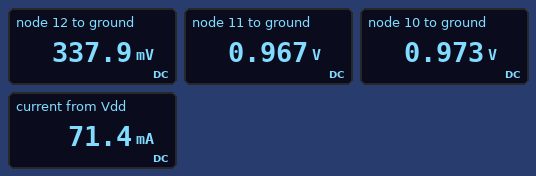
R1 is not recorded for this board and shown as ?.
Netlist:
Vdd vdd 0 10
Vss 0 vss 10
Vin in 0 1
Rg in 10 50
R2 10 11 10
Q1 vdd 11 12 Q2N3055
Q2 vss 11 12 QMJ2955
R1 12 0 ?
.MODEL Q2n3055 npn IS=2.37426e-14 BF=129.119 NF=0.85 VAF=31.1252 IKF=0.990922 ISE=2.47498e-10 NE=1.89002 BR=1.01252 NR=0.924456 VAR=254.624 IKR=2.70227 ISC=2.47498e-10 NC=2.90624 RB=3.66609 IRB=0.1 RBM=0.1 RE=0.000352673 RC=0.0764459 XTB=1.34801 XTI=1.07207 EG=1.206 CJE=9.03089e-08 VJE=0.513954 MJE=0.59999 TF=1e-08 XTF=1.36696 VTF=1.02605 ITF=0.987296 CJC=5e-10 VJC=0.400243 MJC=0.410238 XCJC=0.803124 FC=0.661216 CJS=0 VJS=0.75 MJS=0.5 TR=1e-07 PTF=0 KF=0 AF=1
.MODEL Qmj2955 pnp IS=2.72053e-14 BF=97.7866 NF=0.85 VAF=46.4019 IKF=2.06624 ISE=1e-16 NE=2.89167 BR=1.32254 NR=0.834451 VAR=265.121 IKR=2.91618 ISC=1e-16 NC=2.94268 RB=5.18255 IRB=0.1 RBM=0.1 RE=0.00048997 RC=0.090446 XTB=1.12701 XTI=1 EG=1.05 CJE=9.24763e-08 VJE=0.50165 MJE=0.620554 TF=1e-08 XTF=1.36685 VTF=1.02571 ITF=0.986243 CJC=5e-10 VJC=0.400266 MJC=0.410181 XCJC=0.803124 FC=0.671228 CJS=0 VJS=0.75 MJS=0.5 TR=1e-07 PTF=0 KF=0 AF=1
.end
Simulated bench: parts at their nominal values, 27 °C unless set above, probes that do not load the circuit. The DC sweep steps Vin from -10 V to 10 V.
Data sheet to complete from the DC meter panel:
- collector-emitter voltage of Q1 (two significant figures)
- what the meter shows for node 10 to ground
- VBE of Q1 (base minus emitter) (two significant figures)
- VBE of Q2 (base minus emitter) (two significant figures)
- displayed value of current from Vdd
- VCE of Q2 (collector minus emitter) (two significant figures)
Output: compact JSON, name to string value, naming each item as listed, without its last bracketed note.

{"collector-emitter voltage of Q1": "9.7 V", "what the meter shows for node 10 to ground": "0.973 V", "VBE of Q1 (base minus emitter)": "630 mV", "VBE of Q2 (base minus emitter)": "630 mV", "displayed value of current from Vdd": "71.4 mA", "VCE of Q2 (collector minus emitter)": "-10 V"}
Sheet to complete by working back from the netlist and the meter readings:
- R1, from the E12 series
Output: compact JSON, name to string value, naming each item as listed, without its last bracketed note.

{"R1, from the E12 series": "4.7 Ω"}
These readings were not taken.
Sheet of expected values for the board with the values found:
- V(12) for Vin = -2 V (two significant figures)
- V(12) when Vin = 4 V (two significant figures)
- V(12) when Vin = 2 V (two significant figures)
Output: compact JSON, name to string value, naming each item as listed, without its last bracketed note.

{"V(12) for Vin = -2 V": "-1.2 V", "V(12) when Vin = 4 V": "2.9 V", "V(12) when Vin = 2 V": "1.2 V"}
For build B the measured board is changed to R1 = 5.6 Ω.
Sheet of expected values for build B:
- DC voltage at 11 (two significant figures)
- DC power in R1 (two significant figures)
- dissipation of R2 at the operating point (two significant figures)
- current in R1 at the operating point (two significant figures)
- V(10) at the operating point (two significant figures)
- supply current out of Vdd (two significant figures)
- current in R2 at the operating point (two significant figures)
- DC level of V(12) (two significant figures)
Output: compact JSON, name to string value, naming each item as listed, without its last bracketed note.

{"DC voltage at 11": "970 mV", "DC power in R1": "21 mW", "dissipation of R2 at the operating point": "2.2 µW", "current in R1 at the operating point": "62 mA", "V(10) at the operating point": "980 mV", "supply current out of Vdd": "61 mA", "current in R2 at the operating point": "470 µA", "DC level of V(12)": "350 mV"}
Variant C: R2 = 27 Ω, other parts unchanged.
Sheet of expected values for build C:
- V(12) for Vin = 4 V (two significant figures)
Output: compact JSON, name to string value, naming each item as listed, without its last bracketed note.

{"V(12) for Vin = 4 V": "2.8 V"}
